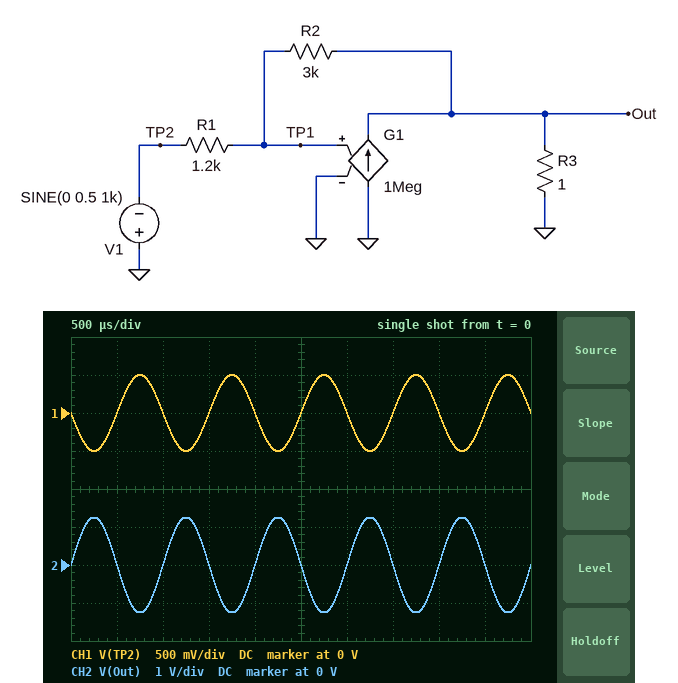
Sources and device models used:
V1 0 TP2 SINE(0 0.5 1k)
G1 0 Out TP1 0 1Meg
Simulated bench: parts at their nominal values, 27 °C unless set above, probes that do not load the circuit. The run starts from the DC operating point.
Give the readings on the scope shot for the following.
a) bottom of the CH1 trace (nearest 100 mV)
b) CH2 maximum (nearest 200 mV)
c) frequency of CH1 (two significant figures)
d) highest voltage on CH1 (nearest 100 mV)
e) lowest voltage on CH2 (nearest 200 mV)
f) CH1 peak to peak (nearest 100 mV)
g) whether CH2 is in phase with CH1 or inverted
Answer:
-500 mV
1.2 V
1.0 kHz
500 mV
-1.2 V
1.0 V
inverted
